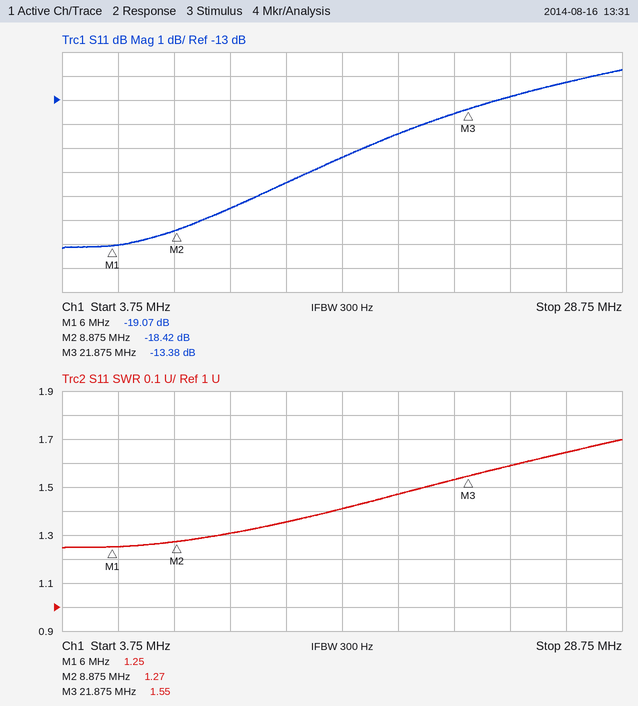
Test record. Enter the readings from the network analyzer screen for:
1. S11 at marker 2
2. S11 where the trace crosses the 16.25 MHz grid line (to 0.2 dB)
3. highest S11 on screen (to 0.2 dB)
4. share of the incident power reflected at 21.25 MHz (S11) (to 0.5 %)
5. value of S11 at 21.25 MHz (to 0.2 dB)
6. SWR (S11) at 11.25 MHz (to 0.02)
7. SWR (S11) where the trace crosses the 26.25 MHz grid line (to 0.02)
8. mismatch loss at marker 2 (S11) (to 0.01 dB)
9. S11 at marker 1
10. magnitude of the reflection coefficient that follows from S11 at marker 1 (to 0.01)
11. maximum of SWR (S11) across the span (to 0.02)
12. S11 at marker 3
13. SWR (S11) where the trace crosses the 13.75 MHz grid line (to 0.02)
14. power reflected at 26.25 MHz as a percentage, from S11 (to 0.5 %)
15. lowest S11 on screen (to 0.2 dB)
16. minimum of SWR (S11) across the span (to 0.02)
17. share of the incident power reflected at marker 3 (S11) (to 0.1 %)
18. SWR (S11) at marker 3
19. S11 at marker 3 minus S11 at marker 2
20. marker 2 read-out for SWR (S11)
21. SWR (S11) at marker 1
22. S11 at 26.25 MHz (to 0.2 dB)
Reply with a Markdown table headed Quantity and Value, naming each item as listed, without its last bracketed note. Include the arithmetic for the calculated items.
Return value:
| Quantity | Value |
|---|---|
| S11 at marker 2 | -18.42 dB |
| S11 where the trace crosses the 16.25 MHz grid line | -15.4 dB |
| highest S11 on screen | -11.8 dB |
| share of the incident power reflected at 21.25 MHz (S11) | 10^(-13.6/10) ≈ 4.37 %, so 4.5 % to the nearest 0.5 % |
| value of S11 at 21.25 MHz | -13.6 dB |
| SWR (S11) at 11.25 MHz | 1.30 |
| SWR (S11) where the trace crosses the 26.25 MHz grid line | 1.64 |
| mismatch loss at marker 2 (S11) | −10 log10(1 − 10^(-18.42/10)) ≈ 0.06 dB |
| S11 at marker 1 | -19.07 dB |
| magnitude of the reflection coefficient that follows from S11 at marker 1 | 10^(-19.07/20) ≈ 0.11 |
| maximum of SWR (S11) across the span | 1.70 |
| S11 at marker 3 | -13.38 dB |
| SWR (S11) where the trace crosses the 13.75 MHz grid line | 1.36 |
| power reflected at 26.25 MHz as a percentage, from S11 | 10^(-12.2/10) ≈ 6.0 % |
| lowest S11 on screen | -19.2 dB |
| minimum of SWR (S11) across the span | 1.24 |
| share of the incident power reflected at marker 3 (S11) | 10^(-13.38/10) ≈ 4.6 % |
| SWR (S11) at marker 3 | 1.55 |
| S11 at marker 3 minus S11 at marker 2 | -13.38 − (-18.42) = 5.04 dB |
| marker 2 read-out for SWR | 1.27 |
| SWR (S11) at marker 1 | 1.25 |
| S11 at 26.25 MHz | -12.2 dB |
